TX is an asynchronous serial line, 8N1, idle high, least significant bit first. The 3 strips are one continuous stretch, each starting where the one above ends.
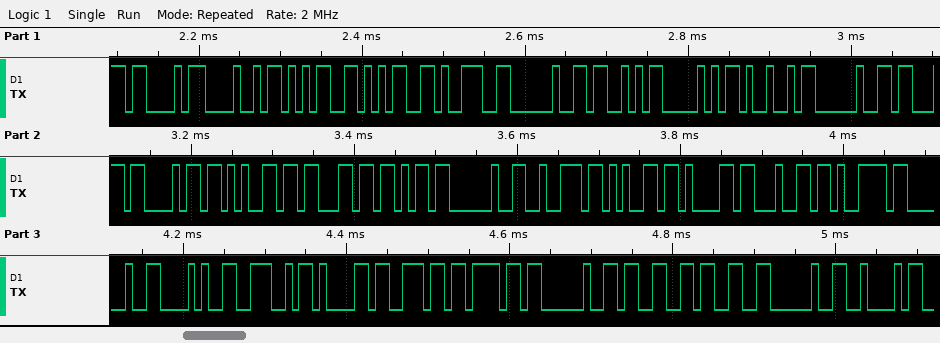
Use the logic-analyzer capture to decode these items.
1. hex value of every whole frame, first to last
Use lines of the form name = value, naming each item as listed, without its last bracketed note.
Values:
hex value of every whole frame, first to last = 0x43 0x48 0x35 0x35 0x39 0x20 0x53 0x50 0x49 0x20 0x63 0x68 0x65 0x63 0x6B 0x20 0x72 0x65 0x61 0x64 0x79 0x20 0x28 0x4E 0x61 0x6E 0x6F 0x20 0x33 0x33 0x20 0x42
